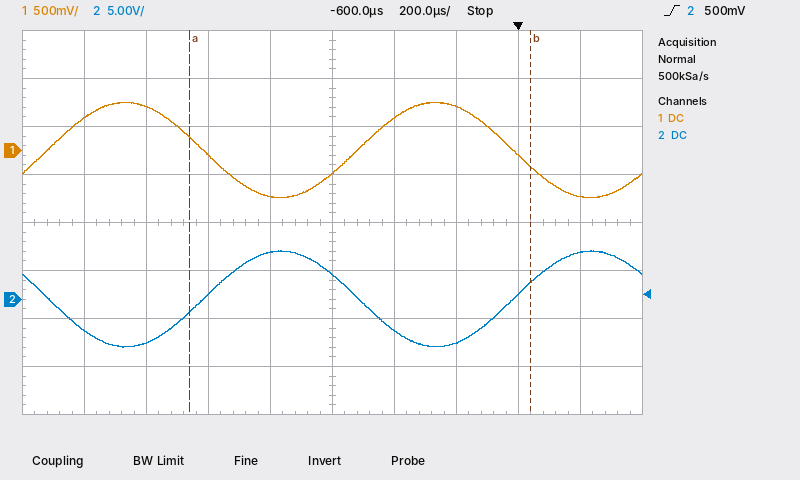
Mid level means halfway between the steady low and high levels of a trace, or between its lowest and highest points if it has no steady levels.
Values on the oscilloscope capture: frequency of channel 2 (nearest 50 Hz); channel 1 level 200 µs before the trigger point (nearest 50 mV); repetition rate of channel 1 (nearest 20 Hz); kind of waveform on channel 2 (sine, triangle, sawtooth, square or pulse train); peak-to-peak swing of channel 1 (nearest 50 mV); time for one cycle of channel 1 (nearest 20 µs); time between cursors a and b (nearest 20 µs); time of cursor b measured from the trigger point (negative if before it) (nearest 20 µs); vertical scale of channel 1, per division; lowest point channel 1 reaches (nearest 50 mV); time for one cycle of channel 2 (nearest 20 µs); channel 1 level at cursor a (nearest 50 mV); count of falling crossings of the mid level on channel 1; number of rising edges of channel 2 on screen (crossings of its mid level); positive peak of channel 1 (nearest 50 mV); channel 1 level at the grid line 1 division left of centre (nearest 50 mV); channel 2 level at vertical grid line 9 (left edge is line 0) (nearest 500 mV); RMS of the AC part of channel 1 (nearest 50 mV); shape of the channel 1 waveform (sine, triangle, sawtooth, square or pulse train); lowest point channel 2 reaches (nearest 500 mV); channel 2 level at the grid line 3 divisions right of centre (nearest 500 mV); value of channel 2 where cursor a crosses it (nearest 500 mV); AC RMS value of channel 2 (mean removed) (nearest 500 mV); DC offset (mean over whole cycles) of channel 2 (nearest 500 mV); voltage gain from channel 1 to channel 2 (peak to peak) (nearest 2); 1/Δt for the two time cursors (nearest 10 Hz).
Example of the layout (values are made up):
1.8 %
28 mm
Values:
1.00 kHz
450 mV
1.00 kHz
sine
1.00 V
1.00 ms
1.10 ms
+40 µs
500 mV
-500 mV
1.00 ms
150 mV
2
2
500 mV
-500 mV
5.0 V
350 mV
sine
-5.0 V
500 mV
-1.5 V
3.5 V
0.0 V
10
910 Hz
